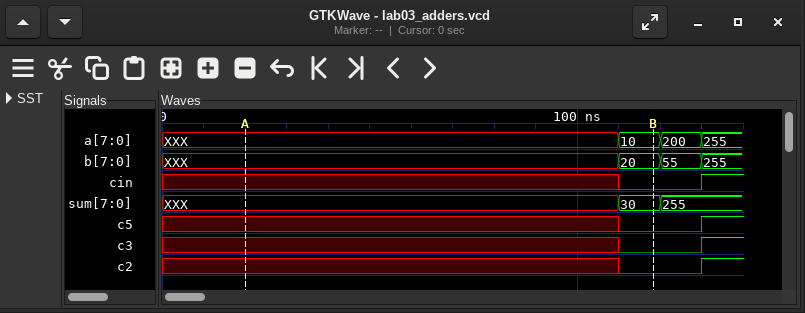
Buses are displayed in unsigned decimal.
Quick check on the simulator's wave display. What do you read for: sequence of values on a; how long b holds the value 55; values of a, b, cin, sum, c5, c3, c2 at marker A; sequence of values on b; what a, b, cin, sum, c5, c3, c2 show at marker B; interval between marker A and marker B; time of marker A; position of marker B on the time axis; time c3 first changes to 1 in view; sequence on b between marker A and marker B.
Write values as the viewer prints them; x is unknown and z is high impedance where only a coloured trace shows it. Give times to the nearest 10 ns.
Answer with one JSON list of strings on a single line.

["XXX, 10, 200, 255", "10 ns", "a=XXX, b=XXX, cin=x, sum=XXX, c5=x, c3=x, c2=x", "XXX, 20, 55, 255", "a=10, b=20, cin=0, sum=30, c5=0, c3=0, c2=0", "100 ns", "20 ns", "120 ns", "130 ns", "XXX, 20"]
